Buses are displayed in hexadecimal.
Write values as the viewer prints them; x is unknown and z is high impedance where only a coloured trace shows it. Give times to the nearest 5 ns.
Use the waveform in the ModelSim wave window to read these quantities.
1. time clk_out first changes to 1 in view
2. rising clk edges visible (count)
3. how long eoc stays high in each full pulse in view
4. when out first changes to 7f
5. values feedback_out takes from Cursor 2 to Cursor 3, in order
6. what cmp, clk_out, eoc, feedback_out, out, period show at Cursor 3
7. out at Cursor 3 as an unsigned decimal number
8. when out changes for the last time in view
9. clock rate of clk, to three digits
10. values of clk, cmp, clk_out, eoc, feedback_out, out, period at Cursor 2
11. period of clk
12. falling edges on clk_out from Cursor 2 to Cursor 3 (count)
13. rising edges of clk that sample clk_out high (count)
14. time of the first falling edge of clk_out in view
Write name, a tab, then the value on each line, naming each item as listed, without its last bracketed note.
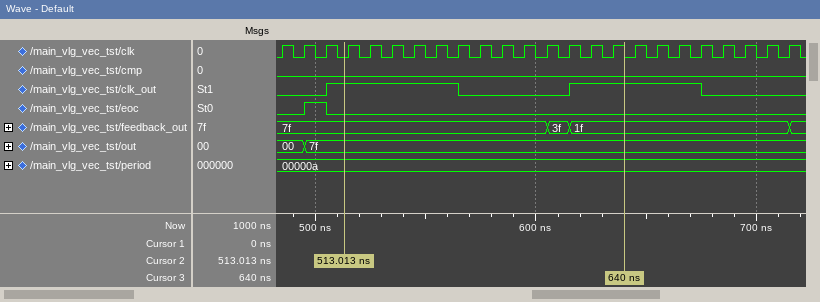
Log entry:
time clk_out first changes to 1 in view	505 ns
rising clk edges visible	24
how long eoc stays high in each full pulse in view	10 ns
when out first changes to 7f	495 ns
values feedback_out takes from Cursor 2 to Cursor 3, in order	7f, 3f, 1f
what cmp, clk_out, eoc, feedback_out, out, period show at Cursor 3	cmp=0, clk_out=1, eoc=0, feedback_out=1f, out=7f, period=00000a
out at Cursor 3 as an unsigned decimal number	127
when out changes for the last time in view	495 ns
clock rate of clk, to three digits	100 MHz
values of clk, cmp, clk_out, eoc, feedback_out, out, period at Cursor 2	clk=0, cmp=0, clk_out=1, eoc=0, feedback_out=7f, out=7f, period=00000a
period of clk	10 ns
falling edges on clk_out from Cursor 2 to Cursor 3	1
rising edges of clk that sample clk_out high	12
time of the first falling edge of clk_out in view	565 ns
